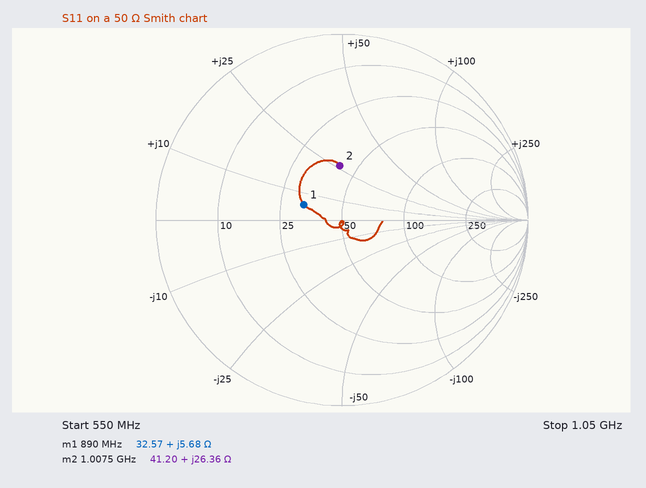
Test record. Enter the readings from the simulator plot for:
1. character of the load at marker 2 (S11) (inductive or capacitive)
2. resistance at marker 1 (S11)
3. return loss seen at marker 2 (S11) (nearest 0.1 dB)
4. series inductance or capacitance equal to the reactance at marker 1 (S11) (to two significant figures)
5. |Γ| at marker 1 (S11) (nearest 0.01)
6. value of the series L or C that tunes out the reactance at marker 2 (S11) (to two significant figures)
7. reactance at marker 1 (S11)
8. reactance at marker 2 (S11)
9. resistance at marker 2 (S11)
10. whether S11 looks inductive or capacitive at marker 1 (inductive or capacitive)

inductive
32.57 Ω
10.7 dB
1.0 nH
0.22
6.0 pF
+5.68 Ω
+26.36 Ω
41.20 Ω
inductive
